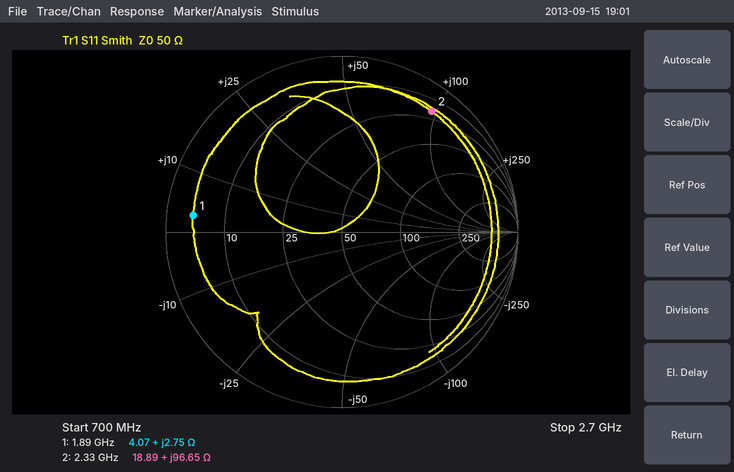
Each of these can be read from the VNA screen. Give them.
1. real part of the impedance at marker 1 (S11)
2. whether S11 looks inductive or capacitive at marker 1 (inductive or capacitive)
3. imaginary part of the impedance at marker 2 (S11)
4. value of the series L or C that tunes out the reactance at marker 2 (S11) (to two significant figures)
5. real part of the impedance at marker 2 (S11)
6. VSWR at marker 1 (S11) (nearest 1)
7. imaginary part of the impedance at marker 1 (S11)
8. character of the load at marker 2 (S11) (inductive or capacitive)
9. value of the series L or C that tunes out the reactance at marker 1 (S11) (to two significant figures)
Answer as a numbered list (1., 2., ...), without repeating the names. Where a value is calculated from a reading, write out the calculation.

1. 4.07 Ω
2. inductive
3. +96.65 Ω
4. C = 1/(2π × 2.33 GHz × 96.65 Ω) ≈ 707 fF, so 710 fF to two significant figures
5. 18.89 Ω
6. 12
7. +2.75 Ω
8. inductive
9. C = 1/(2π × 1.89 GHz × 2.75 Ω) ≈ 31 pF
